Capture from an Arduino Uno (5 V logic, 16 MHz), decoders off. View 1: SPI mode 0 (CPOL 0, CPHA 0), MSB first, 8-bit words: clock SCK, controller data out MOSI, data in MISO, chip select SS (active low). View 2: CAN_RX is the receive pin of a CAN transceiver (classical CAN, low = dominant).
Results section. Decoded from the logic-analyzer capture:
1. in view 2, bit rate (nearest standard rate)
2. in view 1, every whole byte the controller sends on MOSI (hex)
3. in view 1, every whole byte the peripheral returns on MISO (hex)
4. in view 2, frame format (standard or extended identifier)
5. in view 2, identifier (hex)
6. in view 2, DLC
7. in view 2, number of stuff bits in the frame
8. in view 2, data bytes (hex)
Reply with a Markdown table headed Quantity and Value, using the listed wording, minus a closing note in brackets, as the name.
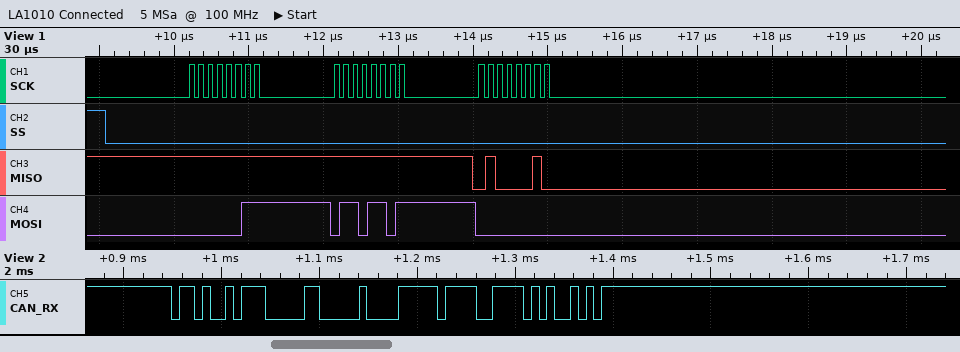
| Quantity | Value |
|---|---|
| in view 2, bit rate | 125 kbit/s |
| in view 1, every whole byte the controller sends on MOSI | 03 6D 00 |
| in view 1, every whole byte the peripheral returns on MISO | FF FF 42 |
| in view 2, frame format | standard |
| in view 2, identifier | 0x697 |
| in view 2, DLC | 2 |
| in view 2, number of stuff bits in the frame | 3 |
| in view 2, data bytes | 00 FF |
